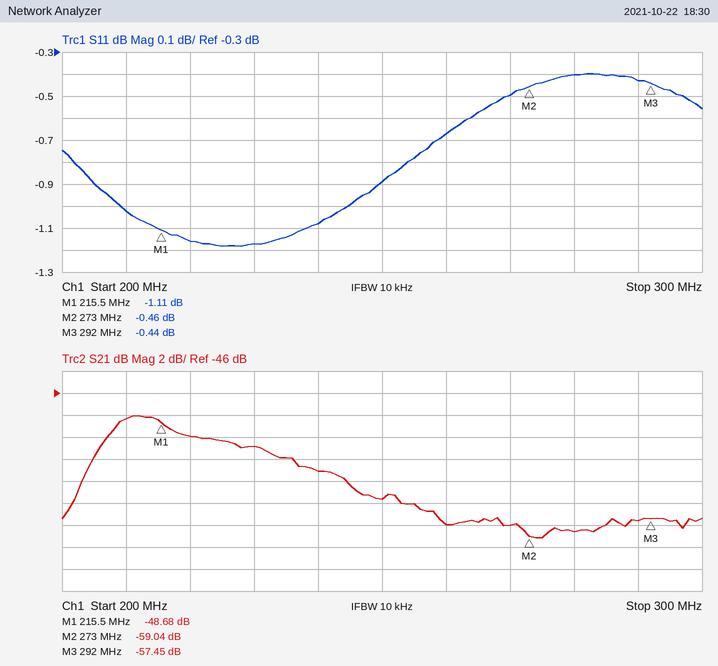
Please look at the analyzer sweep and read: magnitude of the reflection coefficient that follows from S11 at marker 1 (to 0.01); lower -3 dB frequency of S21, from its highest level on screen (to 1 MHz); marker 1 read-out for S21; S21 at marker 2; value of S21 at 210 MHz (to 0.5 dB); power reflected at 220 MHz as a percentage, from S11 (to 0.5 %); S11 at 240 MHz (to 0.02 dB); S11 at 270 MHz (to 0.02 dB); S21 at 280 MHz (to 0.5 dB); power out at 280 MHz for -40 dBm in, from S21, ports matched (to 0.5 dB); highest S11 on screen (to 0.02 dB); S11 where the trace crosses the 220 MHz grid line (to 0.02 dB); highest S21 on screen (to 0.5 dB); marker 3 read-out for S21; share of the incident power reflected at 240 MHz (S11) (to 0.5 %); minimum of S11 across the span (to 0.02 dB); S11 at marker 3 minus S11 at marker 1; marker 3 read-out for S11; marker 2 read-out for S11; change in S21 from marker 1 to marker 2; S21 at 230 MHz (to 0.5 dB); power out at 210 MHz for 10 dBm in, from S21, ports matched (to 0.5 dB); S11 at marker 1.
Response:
0.88
206 MHz
-48.68 dB
-59.04 dB
-48.5 dB
76.5 %
-1.08 dB
-0.50 dB
-58.5 dB
-98.5 dBm
-0.40 dB
-1.16 dB
-48.0 dB
-57.45 dB
78.0 %
-1.18 dB
0.67 dB
-0.44 dB
-0.46 dB
-10.36 dB
-51.0 dB
-38.5 dBm
-1.11 dB
